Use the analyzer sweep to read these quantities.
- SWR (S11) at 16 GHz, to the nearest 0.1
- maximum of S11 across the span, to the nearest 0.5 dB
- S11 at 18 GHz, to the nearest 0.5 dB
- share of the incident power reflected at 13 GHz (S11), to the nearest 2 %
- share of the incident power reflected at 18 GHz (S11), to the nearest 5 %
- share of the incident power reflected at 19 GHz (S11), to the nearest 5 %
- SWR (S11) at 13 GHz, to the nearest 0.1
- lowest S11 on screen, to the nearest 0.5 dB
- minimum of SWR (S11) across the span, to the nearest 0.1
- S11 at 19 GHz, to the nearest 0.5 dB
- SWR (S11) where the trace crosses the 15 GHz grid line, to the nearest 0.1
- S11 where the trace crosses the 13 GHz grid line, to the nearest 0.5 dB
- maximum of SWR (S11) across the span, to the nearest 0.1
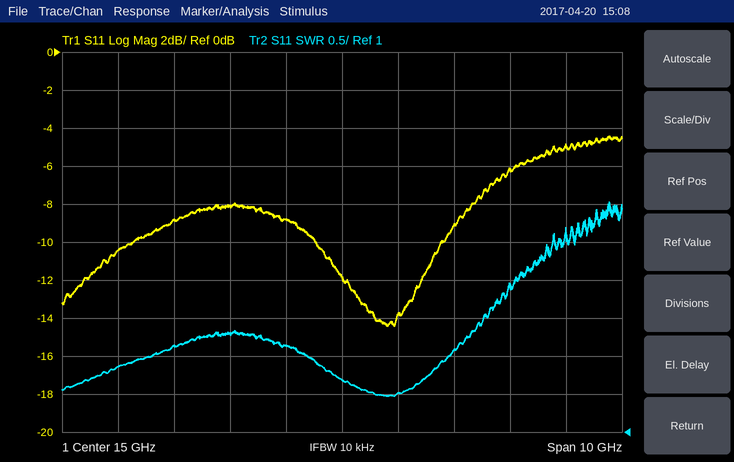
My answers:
1.5
-4.5 dB
-6.0 dB
16 %
25 %
30 %
2.3
-14.5 dB
1.5
-5.0 dB
1.7
-8.0 dB
4.0
